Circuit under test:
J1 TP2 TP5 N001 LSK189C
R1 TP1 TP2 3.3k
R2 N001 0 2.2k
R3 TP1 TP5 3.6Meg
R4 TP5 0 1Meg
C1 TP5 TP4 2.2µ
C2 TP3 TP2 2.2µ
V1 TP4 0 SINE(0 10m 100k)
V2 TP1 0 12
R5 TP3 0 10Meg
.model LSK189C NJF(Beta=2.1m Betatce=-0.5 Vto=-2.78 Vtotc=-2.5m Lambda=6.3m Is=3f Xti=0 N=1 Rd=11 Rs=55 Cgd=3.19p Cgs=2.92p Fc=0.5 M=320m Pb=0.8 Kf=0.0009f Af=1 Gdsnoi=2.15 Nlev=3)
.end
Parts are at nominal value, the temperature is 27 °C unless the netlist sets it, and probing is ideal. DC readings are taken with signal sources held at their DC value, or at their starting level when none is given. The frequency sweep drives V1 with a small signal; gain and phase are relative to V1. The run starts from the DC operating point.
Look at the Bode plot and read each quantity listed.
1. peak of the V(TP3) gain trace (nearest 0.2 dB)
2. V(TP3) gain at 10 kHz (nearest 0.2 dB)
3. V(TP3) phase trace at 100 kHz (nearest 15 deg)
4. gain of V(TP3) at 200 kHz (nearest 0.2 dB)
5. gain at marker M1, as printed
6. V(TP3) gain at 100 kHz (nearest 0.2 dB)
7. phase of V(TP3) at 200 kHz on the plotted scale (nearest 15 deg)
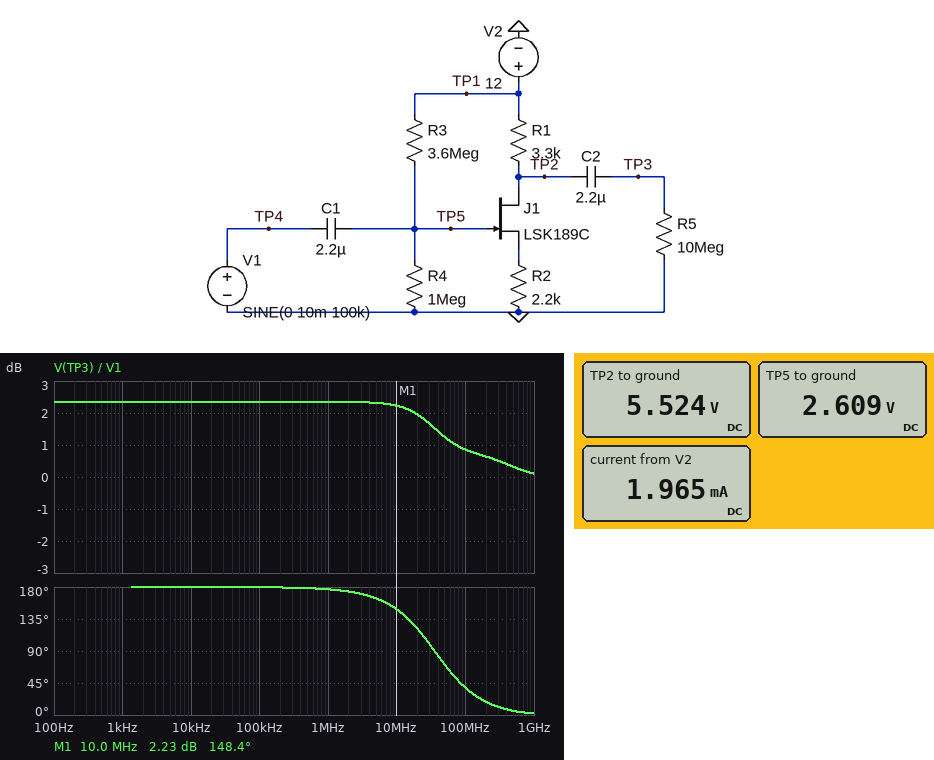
2.4 dB
2.4 dB
180 deg
2.4 dB
2.23 dB
2.4 dB
180 deg
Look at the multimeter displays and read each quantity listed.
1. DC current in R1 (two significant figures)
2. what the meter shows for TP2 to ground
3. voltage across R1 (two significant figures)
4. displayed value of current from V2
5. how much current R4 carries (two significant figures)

2.0 mA
5.524 V
6.5 V
1.965 mA
2.6 µA
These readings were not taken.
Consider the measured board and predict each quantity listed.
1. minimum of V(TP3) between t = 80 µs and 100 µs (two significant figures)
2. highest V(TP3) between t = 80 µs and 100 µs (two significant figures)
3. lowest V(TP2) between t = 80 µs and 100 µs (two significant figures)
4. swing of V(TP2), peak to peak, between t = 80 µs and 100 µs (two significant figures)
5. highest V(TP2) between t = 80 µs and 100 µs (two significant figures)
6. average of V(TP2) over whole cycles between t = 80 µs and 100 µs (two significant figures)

-13 mV
13 mV
5.5 V
26 mV
5.5 V
5.5 V
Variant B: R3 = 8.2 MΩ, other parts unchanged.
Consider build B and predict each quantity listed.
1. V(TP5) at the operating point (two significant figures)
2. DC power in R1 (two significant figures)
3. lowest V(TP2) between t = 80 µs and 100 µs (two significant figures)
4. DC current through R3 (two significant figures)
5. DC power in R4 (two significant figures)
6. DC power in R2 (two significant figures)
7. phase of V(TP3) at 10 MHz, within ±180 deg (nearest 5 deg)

1.3 V
6.9 mW
7.2 V
1.3 µA
1.7 µW
4.6 mW
155 deg
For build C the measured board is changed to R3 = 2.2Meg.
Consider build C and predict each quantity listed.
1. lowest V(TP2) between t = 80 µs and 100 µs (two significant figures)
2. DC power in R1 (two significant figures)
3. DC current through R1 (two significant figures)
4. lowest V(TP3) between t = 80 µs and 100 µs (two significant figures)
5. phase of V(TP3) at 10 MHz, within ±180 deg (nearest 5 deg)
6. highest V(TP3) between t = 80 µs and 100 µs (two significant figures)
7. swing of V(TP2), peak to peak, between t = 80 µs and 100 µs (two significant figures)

5.1 V
15 mW
2.1 mA
-1.1 mV
90 deg
1.1 mV
2.2 mV
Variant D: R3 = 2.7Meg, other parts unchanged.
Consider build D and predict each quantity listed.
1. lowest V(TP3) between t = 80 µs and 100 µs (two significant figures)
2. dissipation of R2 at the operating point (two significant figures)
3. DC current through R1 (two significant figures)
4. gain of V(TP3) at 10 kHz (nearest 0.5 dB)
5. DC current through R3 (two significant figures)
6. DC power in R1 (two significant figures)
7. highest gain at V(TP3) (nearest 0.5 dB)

-2.3 mV
9.5 mW
2.1 mA
-12.5 dB
3.2 µA
14 mW
0 dB
